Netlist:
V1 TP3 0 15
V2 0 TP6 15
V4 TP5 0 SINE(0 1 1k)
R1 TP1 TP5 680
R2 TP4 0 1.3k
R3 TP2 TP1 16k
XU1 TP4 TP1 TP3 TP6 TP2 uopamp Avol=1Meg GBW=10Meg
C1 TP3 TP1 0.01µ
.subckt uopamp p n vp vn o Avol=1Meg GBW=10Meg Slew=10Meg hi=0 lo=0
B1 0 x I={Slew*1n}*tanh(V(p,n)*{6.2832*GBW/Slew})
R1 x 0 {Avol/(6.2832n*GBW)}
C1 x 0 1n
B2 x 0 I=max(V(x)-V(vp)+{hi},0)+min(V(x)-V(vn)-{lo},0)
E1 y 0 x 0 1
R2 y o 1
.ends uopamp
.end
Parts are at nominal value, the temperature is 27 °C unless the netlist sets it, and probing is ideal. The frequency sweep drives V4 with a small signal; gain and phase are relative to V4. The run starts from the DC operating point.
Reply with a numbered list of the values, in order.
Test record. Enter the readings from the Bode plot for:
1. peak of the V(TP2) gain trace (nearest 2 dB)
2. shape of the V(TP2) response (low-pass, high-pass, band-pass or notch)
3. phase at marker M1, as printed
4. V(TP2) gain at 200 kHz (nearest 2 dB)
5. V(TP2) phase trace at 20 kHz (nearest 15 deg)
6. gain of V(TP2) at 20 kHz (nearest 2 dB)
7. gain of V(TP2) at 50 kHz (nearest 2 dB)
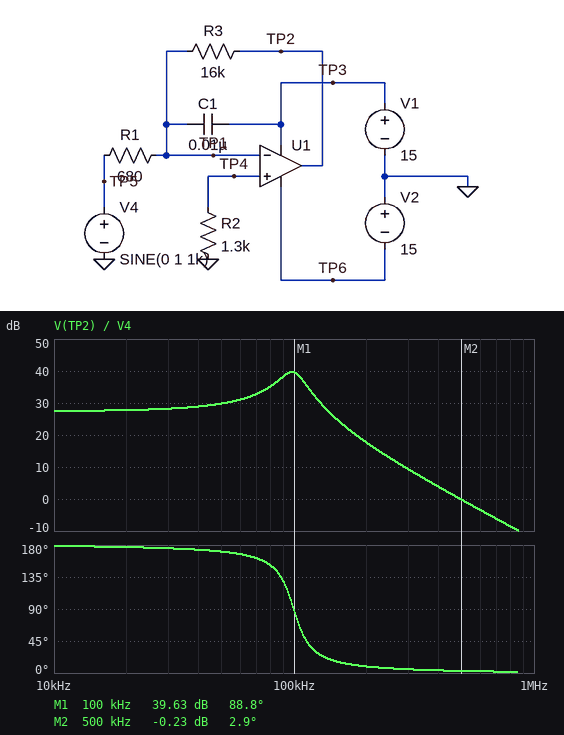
1. 40 dB
2. low-pass
3. 88.8 deg
4. 18 dB
5. 180 deg
6. 28 dB
7. 30 dB
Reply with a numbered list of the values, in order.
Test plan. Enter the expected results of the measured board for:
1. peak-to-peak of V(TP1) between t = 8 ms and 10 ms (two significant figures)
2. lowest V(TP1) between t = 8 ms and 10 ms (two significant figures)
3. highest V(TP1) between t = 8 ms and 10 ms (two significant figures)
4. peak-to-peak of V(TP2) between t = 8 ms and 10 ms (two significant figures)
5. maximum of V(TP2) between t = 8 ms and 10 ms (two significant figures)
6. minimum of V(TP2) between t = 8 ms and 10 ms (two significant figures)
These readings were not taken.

1. 690 mV
2. -350 mV
3. 350 mV
4. 30 V
5. 15 V
6. -15 V
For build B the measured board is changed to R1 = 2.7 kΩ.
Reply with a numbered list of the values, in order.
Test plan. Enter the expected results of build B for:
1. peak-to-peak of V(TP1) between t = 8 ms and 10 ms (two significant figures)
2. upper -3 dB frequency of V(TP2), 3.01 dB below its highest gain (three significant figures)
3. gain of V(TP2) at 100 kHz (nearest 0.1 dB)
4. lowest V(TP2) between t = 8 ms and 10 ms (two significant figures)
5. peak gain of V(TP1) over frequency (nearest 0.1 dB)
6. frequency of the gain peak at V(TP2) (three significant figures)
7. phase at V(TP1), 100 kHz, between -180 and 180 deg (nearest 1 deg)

1. 1.2 mV
2. 103 kHz
3. 38.6 dB
4. -5.9 V
5. -1.4 dB
6. 99.6 kHz
7. -4 deg
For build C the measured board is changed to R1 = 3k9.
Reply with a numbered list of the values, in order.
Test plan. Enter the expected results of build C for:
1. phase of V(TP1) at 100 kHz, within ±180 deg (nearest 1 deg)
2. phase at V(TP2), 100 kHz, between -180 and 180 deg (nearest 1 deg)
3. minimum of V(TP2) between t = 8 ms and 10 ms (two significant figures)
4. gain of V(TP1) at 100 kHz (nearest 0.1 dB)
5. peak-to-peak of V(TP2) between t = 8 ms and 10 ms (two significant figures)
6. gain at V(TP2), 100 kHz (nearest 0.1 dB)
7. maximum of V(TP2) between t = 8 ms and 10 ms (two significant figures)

1. -6 deg
2. 84 deg
3. -4.1 V
4. -2.0 dB
5. 8.2 V
6. 38.0 dB
7. 4.1 V
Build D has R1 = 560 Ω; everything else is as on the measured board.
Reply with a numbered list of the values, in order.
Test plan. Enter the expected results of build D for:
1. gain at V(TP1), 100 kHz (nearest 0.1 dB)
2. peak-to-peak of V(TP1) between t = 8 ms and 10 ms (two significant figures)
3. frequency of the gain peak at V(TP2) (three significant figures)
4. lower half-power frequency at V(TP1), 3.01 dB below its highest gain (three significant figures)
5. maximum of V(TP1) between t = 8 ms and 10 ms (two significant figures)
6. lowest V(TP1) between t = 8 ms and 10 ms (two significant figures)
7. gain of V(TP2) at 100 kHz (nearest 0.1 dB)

1. -0.3 dB
2. 920 mV
3. 97.5 kHz
4. 86.1 kHz
5. 460 mV
6. -460 mV
7. 39.7 dB
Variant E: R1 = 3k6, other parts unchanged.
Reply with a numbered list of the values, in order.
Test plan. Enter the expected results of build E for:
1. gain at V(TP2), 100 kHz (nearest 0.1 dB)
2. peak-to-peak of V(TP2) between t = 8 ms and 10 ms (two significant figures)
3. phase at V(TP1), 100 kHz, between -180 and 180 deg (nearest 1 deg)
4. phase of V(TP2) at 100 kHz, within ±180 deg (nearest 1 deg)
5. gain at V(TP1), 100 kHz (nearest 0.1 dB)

1. 38.2 dB
2. 8.9 V
3. -6 deg
4. 84 deg
5. -1.8 dB
